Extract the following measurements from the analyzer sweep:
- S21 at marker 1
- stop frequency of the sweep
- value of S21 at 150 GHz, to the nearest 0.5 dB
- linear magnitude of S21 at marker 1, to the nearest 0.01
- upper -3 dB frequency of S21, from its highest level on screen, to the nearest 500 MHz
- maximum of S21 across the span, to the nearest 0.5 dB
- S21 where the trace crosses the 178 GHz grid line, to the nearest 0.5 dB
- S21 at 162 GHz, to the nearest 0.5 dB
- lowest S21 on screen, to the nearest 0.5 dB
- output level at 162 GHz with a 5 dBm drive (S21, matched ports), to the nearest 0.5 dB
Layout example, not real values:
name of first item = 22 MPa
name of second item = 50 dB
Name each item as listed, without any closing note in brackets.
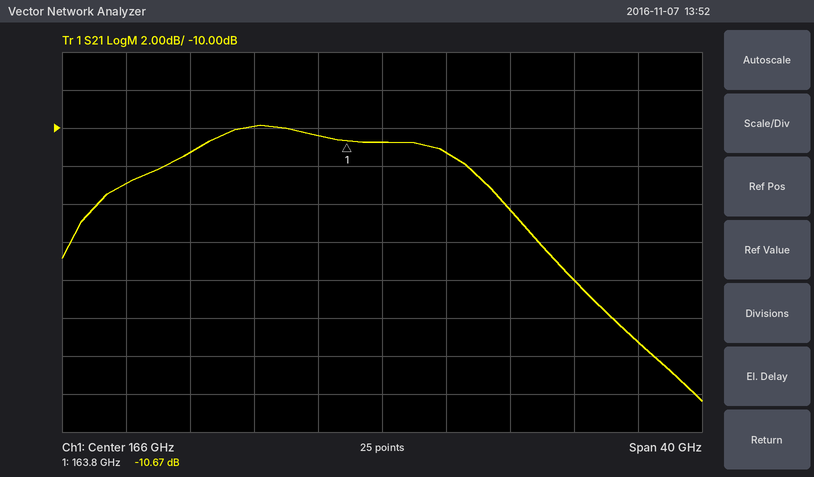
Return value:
S21 at marker 1 = -10.67 dB
stop frequency of the sweep = 186 GHz
value of S21 at 150 GHz, to the nearest 0.5 dB = -13.0 dB
linear magnitude of S21 at marker 1, to the nearest 0.01 = 0.29
upper -3 dB frequency of S21, from its highest level on screen, to the nearest 500 MHz = 172.5 GHz
maximum of S21 across the span, to the nearest 0.5 dB = -10.0 dB
S21 where the trace crosses the 178 GHz grid line, to the nearest 0.5 dB = -18.0 dB
S21 at 162 GHz, to the nearest 0.5 dB = -10.5 dB
lowest S21 on screen, to the nearest 0.5 dB = -24.5 dB
output level at 162 GHz with a 5 dBm drive (S21, matched ports), to the nearest 0.5 dB = -5.5 dBm
